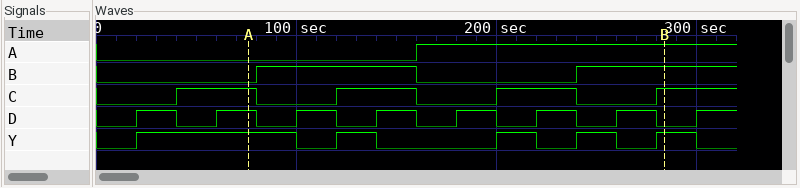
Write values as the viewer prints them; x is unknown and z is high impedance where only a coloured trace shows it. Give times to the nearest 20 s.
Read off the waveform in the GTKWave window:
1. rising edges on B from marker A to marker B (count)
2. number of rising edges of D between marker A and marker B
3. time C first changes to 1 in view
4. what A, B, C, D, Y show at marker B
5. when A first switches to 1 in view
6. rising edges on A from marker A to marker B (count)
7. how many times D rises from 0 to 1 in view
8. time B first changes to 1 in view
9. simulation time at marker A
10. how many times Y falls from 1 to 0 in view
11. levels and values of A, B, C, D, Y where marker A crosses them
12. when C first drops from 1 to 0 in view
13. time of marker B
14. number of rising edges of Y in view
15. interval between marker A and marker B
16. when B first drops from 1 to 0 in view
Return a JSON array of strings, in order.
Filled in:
["2", "5", "40 s", "A=1, B=1, C=1, D=0, Y=1", "160 s", "1", "8", "80 s", "80 s", "5", "A=0, B=0, C=1, D=1, Y=1", "80 s", "280 s", "5", "200 s", "160 s"]
